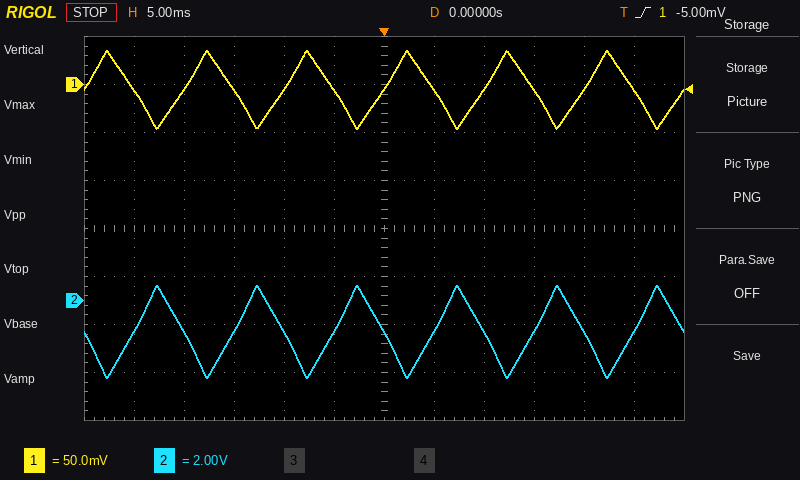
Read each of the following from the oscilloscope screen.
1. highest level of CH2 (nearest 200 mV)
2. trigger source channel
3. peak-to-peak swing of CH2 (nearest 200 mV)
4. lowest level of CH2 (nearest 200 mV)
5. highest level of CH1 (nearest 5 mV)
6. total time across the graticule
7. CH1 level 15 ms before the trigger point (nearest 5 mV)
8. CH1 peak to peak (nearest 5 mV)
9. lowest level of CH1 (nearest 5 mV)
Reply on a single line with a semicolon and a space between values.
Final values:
600 mV; CH1; 3.8 V; -3.2 V; 35 mV; 60 ms; -5 mV; 80 mV; -45 mV
